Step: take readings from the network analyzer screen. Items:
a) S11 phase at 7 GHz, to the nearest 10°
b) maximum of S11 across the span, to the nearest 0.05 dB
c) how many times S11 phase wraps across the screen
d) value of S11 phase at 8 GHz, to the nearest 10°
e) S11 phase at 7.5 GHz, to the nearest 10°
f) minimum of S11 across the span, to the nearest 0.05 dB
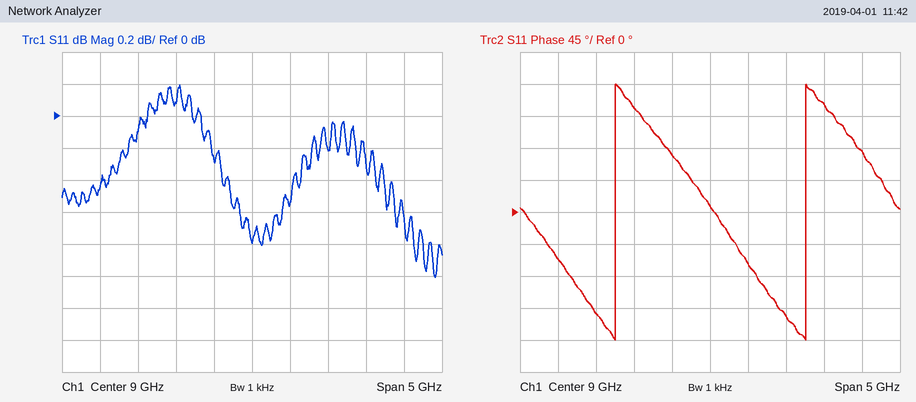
-70°
0.20 dB
2
150°
-140°
-1.00 dB
